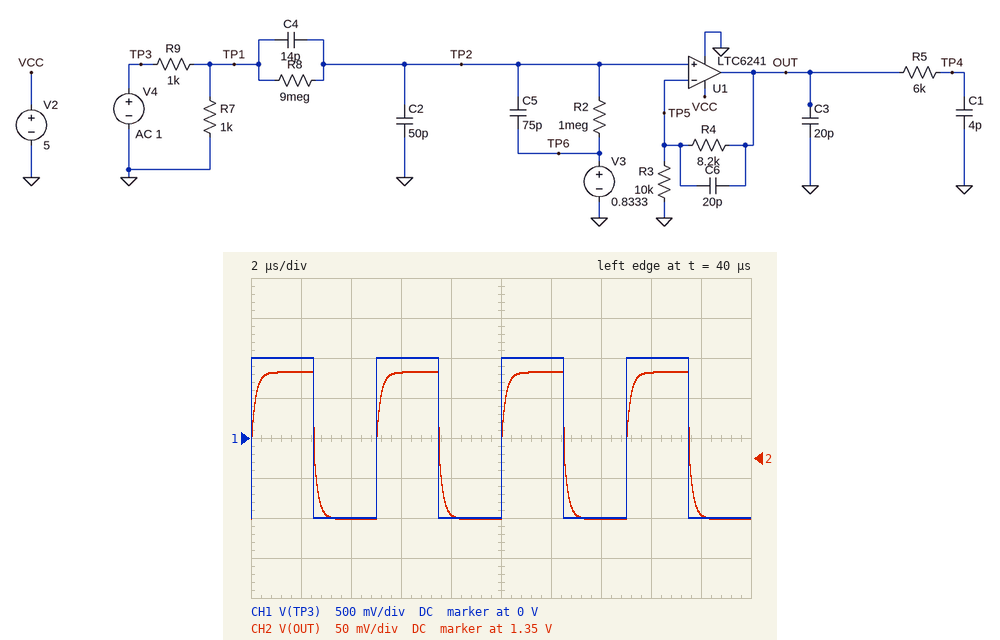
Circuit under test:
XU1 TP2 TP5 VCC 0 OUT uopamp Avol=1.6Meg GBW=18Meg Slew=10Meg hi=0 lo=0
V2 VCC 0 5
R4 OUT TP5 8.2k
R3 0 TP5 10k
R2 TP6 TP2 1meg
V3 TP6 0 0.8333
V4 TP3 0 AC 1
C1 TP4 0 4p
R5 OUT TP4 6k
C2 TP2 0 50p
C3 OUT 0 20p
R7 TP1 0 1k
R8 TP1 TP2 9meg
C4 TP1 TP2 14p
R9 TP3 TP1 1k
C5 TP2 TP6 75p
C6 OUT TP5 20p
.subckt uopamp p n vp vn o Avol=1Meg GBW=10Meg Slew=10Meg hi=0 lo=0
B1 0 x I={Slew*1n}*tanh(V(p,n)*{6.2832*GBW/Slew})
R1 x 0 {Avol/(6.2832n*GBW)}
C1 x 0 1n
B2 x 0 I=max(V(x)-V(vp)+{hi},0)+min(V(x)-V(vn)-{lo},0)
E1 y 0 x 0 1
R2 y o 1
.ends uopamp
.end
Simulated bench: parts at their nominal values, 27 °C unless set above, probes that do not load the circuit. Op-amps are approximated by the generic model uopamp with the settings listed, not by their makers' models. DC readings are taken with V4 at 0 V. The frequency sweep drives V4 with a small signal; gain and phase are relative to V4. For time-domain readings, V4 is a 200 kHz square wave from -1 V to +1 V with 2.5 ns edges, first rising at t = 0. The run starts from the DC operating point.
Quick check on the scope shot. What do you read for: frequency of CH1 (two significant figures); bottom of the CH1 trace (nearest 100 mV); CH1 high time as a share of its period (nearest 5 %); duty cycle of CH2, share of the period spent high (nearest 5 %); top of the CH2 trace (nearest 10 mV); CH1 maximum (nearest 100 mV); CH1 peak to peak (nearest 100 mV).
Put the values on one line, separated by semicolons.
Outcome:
200 kHz; -1.0 V; 50 %; 50 %; 1.46 V; 1.0 V; 2.0 V
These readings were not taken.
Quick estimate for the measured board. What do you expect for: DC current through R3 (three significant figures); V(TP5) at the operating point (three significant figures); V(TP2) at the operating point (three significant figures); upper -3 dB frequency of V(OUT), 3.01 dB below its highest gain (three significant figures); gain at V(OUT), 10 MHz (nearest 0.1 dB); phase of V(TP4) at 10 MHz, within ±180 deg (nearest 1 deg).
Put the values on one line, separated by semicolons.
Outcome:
75.0 µA; 750 mV; 750 mV; 1.37 MHz; -28.0 dB; -111 deg
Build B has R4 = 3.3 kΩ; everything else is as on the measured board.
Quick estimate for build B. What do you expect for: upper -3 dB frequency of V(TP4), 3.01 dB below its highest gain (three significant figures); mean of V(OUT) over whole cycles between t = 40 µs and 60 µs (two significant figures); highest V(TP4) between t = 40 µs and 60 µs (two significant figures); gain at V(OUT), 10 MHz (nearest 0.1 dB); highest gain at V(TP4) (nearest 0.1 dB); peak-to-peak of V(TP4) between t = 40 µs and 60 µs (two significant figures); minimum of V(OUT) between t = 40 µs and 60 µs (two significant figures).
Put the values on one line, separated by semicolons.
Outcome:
3.41 MHz; 1.0 V; 1.1 V; -27.9 dB; -23.5 dB; 130 mV; 930 mV
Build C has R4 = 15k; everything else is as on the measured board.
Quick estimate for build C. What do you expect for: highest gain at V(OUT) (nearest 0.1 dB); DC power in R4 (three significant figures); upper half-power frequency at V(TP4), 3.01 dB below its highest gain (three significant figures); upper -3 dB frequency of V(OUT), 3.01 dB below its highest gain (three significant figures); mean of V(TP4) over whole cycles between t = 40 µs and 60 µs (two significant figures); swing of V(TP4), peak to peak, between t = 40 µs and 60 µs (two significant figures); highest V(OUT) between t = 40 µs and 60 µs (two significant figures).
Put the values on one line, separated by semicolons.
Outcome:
-18.0 dB; 84.4 µW; 597 kHz; 603 kHz; 1.9 V; 250 mV; 2.0 V
